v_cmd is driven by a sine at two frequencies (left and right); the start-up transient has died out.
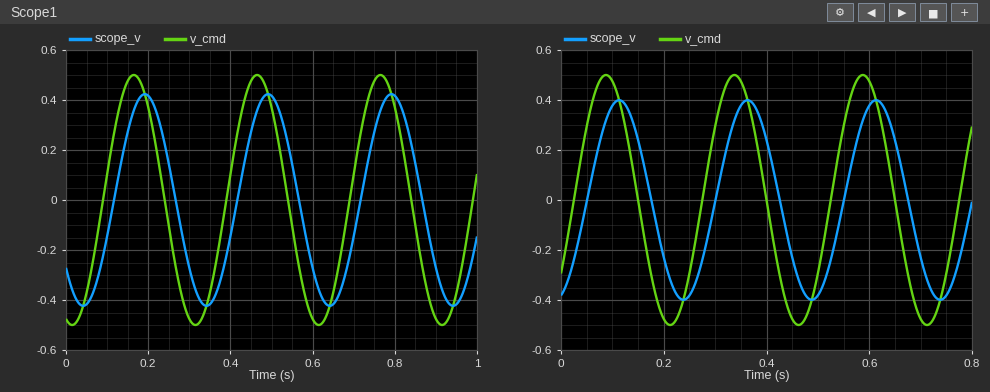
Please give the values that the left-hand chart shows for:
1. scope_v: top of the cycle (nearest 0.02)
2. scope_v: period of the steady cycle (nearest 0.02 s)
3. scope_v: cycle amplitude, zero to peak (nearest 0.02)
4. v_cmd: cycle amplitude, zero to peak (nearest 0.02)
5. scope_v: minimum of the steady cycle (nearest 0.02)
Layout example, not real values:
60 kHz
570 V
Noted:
0.42
0.30 s
0.42
0.50
-0.42
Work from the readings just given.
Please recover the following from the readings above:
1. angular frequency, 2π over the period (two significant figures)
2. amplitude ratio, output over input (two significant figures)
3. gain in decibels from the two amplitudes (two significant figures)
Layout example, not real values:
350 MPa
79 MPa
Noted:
21 rad/s
0.84
-1.5 dB
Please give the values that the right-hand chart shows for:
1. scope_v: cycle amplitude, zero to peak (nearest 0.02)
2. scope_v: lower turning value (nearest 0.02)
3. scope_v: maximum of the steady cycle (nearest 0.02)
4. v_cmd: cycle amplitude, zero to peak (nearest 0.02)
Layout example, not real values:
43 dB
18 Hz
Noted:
0.40
-0.40
0.40
0.50
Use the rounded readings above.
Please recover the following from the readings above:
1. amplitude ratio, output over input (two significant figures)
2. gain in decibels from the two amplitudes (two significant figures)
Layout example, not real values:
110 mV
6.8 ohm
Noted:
0.80
-1.9 dB
